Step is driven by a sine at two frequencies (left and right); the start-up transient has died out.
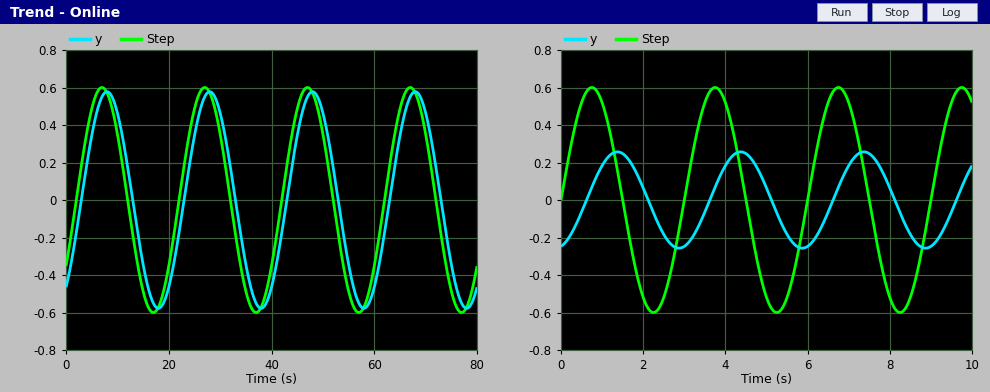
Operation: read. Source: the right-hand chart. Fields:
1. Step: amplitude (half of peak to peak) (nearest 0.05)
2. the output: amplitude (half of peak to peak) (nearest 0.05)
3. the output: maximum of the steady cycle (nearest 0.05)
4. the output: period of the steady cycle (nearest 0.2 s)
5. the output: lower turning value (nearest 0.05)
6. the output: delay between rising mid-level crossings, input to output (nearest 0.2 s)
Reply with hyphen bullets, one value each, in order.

- 0.60
- 0.25
- 0.25
- 3.0 s
- -0.25
- 0.6 s
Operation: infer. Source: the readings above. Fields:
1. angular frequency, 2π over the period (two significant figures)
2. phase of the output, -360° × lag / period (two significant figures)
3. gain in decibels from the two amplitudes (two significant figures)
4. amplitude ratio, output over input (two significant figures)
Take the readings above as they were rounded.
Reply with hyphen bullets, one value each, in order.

- 2.1 rad/s
- -72°
- -7.6 dB
- 0.42
